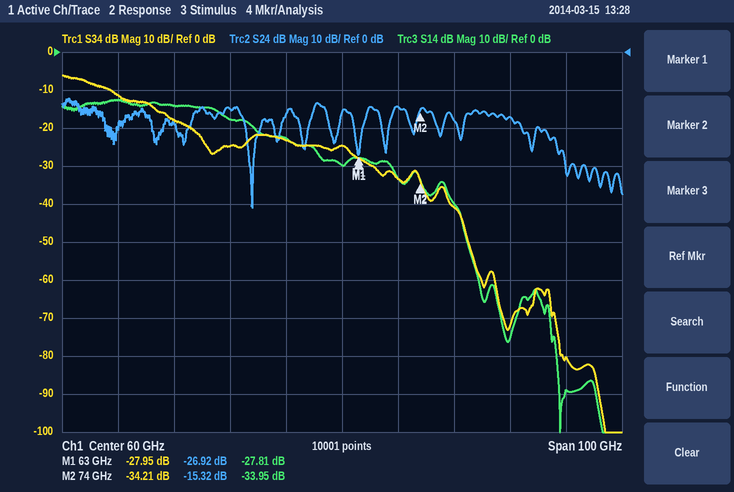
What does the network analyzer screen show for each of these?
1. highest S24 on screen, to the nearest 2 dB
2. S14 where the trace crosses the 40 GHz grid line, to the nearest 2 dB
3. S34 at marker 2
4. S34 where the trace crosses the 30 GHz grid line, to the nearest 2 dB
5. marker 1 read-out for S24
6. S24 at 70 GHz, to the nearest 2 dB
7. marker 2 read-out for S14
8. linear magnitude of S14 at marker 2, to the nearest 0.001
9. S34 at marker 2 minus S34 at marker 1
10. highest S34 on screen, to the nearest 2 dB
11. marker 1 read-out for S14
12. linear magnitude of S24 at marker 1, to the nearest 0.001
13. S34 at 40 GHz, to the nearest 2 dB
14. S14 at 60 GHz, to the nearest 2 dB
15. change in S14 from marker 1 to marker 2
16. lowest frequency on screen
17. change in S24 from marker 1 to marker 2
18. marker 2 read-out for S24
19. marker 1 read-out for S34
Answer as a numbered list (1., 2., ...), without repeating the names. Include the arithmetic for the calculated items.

1. -12 dB
2. -18 dB
3. -34.21 dB
4. -18 dB
5. -26.92 dB
6. -14 dB
7. -33.95 dB
8. 10^(-33.95/20) ≈ 0.020
9. -34.21 − (-27.95) = -6.26 dB
10. -6 dB
11. -27.81 dB
12. 10^(-26.92/20) ≈ 0.045
13. -24 dB
14. -30 dB
15. -33.95 − (-27.81) = -6.14 dB
16. 10 GHz
17. -15.32 − (-26.92) = 11.60 dB
18. -15.32 dB
19. -27.95 dB
